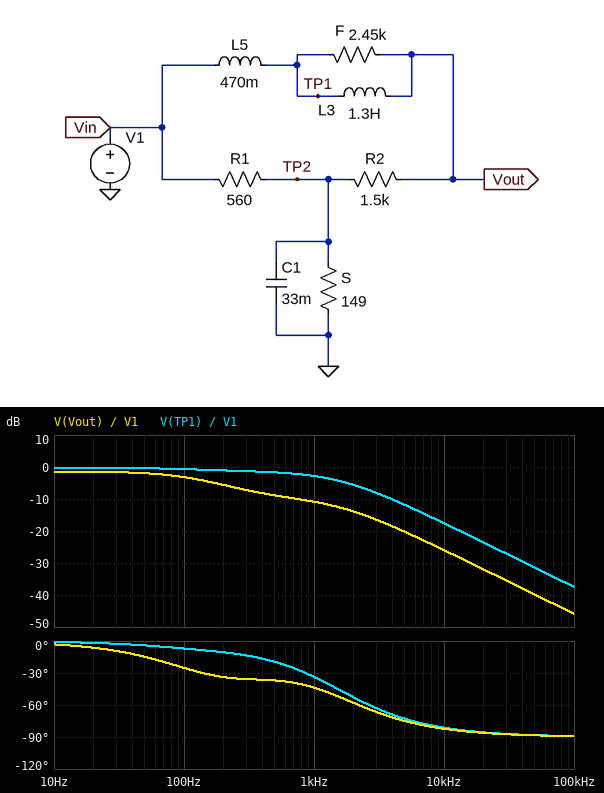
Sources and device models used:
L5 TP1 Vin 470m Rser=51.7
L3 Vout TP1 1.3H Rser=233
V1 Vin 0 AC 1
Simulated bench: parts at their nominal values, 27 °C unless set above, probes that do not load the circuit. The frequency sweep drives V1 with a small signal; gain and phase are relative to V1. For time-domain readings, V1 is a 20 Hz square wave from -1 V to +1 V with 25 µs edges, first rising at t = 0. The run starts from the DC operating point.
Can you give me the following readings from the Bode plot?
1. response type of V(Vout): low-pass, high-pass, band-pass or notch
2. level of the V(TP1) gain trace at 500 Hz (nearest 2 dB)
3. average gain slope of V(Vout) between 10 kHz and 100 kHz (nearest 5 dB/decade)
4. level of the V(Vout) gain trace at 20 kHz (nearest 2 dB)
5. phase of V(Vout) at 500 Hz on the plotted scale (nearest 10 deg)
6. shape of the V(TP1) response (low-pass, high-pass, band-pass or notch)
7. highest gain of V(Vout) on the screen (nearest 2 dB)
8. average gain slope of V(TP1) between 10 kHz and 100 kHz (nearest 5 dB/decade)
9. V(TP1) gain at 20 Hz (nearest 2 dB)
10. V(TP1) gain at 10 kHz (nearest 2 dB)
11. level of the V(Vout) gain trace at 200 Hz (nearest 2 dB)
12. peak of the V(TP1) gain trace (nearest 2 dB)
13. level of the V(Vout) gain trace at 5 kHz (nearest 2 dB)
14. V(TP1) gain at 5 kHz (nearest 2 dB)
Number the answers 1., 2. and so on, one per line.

1. low-pass
2. -2 dB
3. -20 dB/decade
4. -32 dB
5. -40 deg
6. low-pass
7. -2 dB
8. -20 dB/decade
9. 0 dB
10. -18 dB
11. -6 dB
12. 0 dB
13. -20 dB
14. -12 dB
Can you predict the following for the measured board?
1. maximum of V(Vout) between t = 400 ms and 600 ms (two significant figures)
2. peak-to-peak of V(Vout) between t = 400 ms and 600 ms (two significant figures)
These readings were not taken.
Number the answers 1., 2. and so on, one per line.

1. 820 mV
2. 1.7 V
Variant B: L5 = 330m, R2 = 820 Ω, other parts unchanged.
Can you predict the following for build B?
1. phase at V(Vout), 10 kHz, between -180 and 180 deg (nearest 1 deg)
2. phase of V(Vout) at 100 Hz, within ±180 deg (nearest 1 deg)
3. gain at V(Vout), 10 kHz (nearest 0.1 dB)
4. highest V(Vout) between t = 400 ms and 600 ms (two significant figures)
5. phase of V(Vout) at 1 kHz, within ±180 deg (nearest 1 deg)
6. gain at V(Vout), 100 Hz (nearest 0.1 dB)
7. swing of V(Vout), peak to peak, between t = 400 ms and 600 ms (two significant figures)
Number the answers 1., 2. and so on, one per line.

1. -81 deg
2. -33 deg
3. -28.2 dB
4. 700 mV
5. -41 deg
6. -5.4 dB
7. 1.5 V
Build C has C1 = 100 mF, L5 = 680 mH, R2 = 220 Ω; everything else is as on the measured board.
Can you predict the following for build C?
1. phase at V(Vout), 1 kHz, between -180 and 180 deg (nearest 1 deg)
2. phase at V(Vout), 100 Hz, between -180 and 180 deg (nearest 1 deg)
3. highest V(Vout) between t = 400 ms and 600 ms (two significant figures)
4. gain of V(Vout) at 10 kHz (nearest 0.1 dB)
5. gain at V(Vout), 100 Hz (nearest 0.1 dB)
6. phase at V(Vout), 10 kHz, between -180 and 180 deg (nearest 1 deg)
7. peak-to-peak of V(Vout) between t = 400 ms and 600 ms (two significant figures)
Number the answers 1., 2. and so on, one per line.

1. -63 deg
2. -57 deg
3. 270 mV
4. -45.8 dB
5. -15.1 dB
6. -86 deg
7. 910 mV
